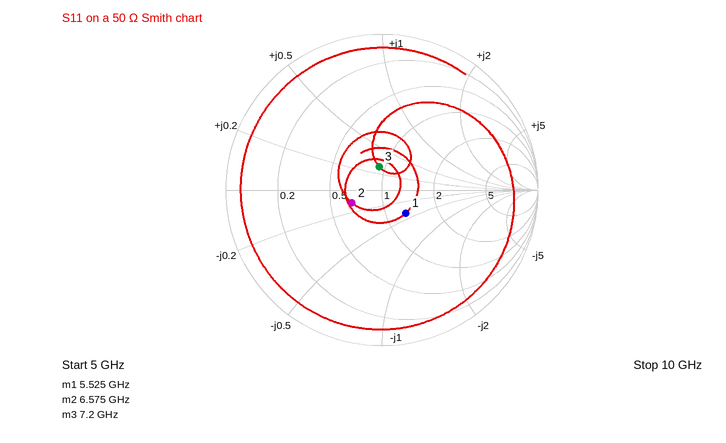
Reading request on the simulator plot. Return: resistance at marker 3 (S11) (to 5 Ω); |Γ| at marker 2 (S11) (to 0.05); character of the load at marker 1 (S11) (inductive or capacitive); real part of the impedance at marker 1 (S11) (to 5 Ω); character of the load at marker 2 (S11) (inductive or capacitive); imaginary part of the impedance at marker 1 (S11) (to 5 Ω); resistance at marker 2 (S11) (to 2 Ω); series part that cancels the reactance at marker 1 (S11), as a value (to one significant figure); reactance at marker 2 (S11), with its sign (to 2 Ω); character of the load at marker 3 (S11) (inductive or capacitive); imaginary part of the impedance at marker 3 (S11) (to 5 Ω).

45 Ω
0.20
capacitive
65 Ω
capacitive
-20 Ω
34 Ω
600 pH
-6 Ω
inductive
+15 Ω
